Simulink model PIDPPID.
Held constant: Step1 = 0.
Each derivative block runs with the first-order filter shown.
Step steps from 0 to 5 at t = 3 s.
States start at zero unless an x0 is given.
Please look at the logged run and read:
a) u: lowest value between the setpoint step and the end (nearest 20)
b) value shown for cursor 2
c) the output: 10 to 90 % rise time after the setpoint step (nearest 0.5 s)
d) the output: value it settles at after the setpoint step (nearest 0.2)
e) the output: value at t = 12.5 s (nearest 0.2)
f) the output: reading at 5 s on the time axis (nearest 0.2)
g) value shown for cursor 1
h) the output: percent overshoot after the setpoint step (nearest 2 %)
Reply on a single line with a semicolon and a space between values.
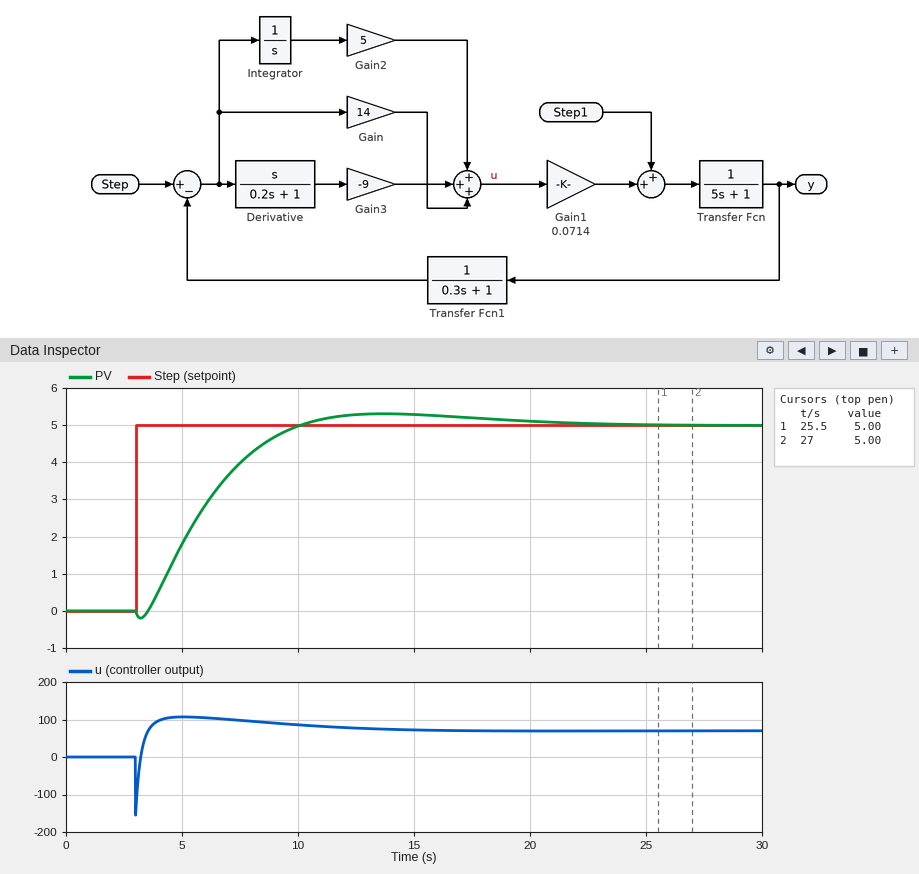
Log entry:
-160; 5.00; 4.5 s; 5.0; 5.2; 1.8; 5.00; 6 %
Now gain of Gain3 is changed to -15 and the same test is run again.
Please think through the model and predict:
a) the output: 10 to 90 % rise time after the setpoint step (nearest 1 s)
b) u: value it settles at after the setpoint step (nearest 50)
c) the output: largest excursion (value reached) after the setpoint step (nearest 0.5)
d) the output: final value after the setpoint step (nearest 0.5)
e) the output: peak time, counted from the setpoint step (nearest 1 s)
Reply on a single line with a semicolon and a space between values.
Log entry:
4 s; 50; 5.5; 5.0; 10 s
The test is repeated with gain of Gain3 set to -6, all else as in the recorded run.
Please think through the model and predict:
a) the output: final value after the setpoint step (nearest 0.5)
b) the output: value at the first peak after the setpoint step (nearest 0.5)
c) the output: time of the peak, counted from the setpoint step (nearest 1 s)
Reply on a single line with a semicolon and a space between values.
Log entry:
5.0; 5.5; 11 s
